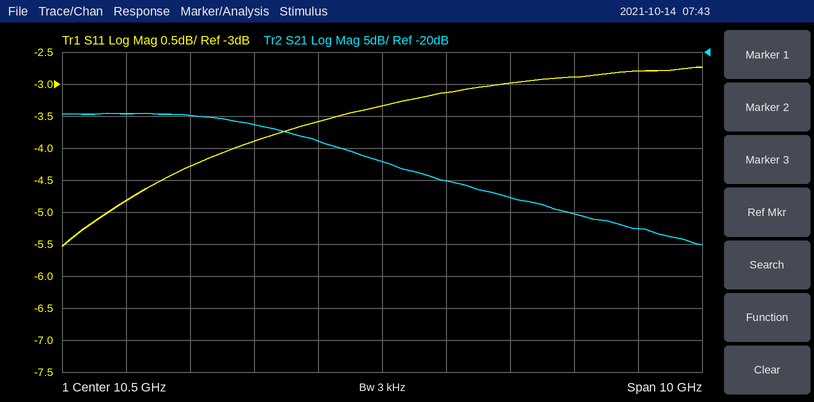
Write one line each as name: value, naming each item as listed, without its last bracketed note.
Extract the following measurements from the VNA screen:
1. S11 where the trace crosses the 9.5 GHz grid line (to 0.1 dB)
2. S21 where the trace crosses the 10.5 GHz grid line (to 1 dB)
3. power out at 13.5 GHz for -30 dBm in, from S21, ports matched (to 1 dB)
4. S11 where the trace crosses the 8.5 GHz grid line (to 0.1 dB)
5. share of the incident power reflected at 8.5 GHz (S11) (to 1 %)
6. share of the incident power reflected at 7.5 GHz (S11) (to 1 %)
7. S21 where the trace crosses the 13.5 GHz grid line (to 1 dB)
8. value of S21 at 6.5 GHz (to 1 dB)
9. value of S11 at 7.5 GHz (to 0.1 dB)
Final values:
S11 where the trace crosses the 9.5 GHz grid line: -3.6 dB
S21 where the trace crosses the 10.5 GHz grid line: -37 dB
power out at 13.5 GHz for -30 dBm in, from S21, ports matched: -75 dBm
S11 where the trace crosses the 8.5 GHz grid line: -3.9 dB
share of the incident power reflected at 8.5 GHz (S11): 41 %
share of the incident power reflected at 7.5 GHz (S11): 37 %
S21 where the trace crosses the 13.5 GHz grid line: -45 dB
value of S21 at 6.5 GHz: -30 dB
value of S11 at 7.5 GHz: -4.3 dB
